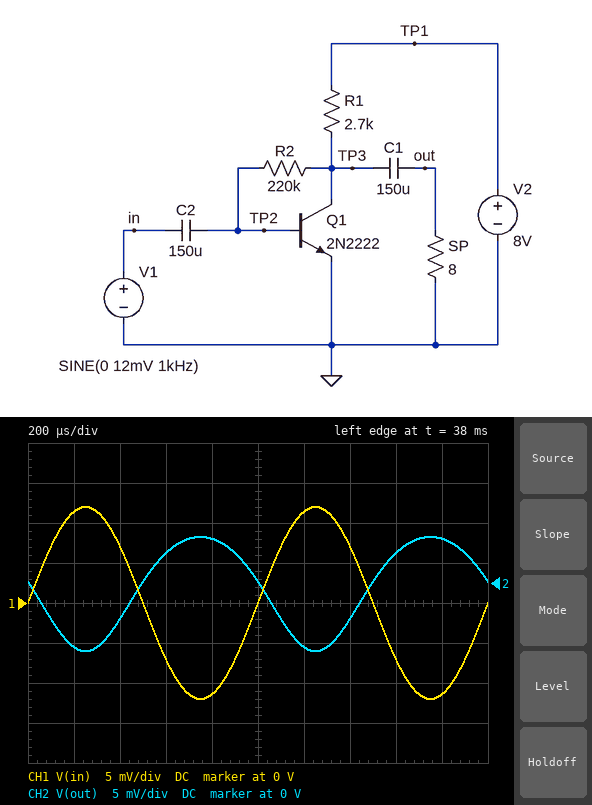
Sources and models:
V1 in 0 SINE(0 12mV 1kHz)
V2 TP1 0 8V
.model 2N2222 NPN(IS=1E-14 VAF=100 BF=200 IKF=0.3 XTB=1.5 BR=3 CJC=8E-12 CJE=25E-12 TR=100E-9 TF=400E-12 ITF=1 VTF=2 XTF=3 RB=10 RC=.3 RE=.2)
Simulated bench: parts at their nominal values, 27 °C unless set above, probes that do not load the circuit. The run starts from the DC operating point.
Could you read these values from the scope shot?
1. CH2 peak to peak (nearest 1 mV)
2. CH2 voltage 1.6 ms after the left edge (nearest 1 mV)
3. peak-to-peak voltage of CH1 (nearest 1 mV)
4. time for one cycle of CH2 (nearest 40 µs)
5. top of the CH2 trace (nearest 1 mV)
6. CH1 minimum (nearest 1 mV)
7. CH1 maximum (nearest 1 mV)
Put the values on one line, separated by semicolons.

14 mV; 4 mV; 24 mV; 1.00 ms; 6 mV; -12 mV; 12 mV
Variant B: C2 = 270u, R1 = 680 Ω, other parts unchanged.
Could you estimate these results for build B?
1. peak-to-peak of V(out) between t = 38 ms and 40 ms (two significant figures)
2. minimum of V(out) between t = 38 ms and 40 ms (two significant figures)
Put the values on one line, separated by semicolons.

30 mV; -17 mV
